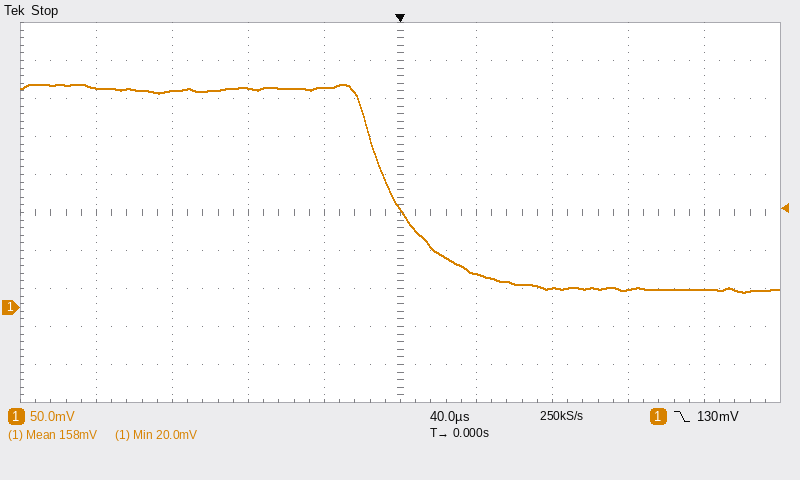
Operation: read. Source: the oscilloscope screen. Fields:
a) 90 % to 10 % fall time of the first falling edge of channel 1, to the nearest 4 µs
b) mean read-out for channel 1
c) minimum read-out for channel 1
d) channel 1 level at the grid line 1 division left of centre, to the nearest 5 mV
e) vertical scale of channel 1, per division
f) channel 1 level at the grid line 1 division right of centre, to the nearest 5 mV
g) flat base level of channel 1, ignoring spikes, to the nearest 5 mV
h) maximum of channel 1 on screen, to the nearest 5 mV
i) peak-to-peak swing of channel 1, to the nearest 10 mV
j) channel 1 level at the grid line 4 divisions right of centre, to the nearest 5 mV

56 µs
158 mV
20.0 mV
290 mV
50 mV
45 mV
25 mV
295 mV
270 mV
25 mV
